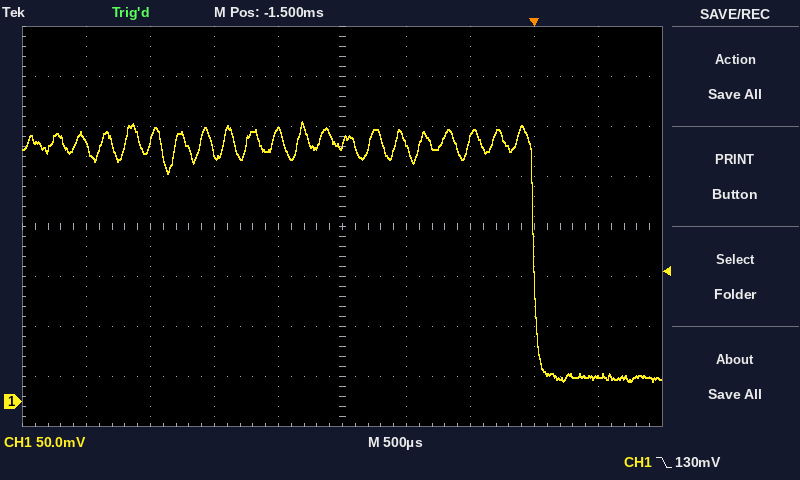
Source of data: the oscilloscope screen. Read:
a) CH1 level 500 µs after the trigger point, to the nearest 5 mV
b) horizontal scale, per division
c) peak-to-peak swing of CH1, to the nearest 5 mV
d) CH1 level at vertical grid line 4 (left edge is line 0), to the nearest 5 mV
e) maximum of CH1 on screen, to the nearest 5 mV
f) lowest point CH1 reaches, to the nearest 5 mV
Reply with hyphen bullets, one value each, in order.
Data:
- 25 mV
- 500 µs
- 260 mV
- 270 mV
- 280 mV
- 20 mV
